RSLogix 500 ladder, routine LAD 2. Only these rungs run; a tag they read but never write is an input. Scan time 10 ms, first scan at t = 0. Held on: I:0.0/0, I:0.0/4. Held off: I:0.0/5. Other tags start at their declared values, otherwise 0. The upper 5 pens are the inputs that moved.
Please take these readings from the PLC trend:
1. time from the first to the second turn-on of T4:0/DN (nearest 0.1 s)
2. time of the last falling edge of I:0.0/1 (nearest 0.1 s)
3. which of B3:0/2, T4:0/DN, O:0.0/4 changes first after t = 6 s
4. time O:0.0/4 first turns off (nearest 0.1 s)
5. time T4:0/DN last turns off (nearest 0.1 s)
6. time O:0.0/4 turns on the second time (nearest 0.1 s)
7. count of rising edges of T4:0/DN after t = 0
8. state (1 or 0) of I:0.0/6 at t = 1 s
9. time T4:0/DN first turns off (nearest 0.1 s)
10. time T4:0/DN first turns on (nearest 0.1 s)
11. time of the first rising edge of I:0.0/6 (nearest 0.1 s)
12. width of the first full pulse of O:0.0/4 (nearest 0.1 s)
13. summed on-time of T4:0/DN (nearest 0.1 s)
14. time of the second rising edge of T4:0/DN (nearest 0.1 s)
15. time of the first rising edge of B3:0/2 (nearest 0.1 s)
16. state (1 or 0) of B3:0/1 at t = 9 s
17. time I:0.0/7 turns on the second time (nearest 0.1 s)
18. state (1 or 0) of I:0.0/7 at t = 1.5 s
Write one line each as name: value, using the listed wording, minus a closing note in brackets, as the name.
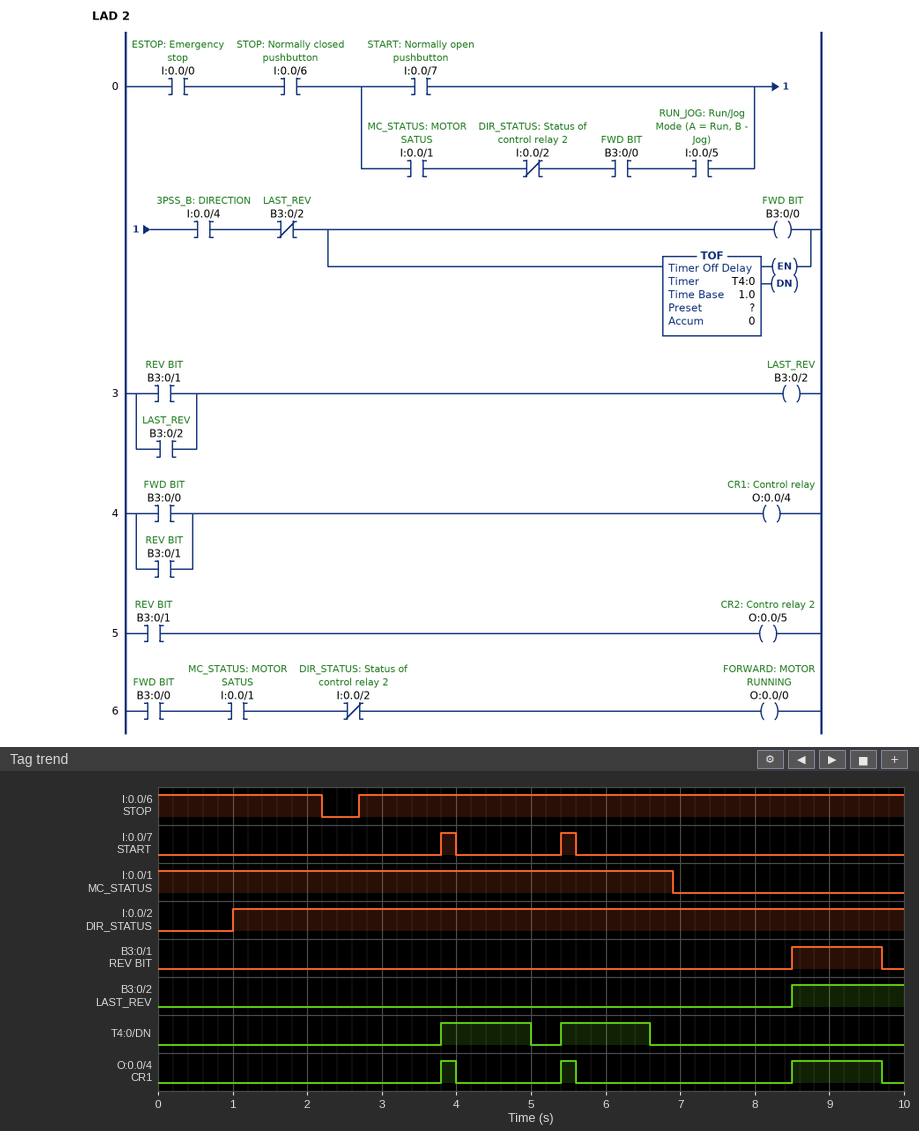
time from the first to the second turn-on of T4:0/DN: 1.6 s
time of the last falling edge of I:0.0/1: 6.9 s
which of B3:0/2, T4:0/DN, O:0.0/4 changes first after t = 6 s: T4:0/DN
time O:0.0/4 first turns off: 4.0 s
time T4:0/DN last turns off: 6.6 s
time O:0.0/4 turns on the second time: 5.4 s
count of rising edges of T4:0/DN after t = 0: 2
state (1 or 0) of I:0.0/6 at t = 1 s: 1
time T4:0/DN first turns off: 5.0 s
time T4:0/DN first turns on: 3.8 s
time of the first rising edge of I:0.0/6: 2.7 s
width of the first full pulse of O:0.0/4: 0.2 s
summed on-time of T4:0/DN: 2.4 s
time of the second rising edge of T4:0/DN: 5.4 s
time of the first rising edge of B3:0/2: 8.5 s
state (1 or 0) of B3:0/1 at t = 9 s: 1
time I:0.0/7 turns on the second time: 5.4 s
state (1 or 0) of I:0.0/7 at t = 1.5 s: 0
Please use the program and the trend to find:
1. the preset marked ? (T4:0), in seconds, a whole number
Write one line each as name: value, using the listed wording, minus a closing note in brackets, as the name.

the preset marked ? (T4:0), in seconds, a whole number: 1 s
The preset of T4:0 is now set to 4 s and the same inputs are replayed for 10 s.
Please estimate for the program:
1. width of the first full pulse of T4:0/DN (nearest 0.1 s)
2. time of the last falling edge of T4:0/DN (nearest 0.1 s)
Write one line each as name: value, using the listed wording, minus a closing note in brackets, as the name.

width of the first full pulse of T4:0/DN: 5.8 s
time of the last falling edge of T4:0/DN: 9.6 s
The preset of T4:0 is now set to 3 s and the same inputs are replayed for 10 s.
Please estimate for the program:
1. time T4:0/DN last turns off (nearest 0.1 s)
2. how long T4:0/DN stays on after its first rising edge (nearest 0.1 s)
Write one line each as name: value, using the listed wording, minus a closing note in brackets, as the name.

time T4:0/DN last turns off: 8.6 s
how long T4:0/DN stays on after its first rising edge: 4.8 s
